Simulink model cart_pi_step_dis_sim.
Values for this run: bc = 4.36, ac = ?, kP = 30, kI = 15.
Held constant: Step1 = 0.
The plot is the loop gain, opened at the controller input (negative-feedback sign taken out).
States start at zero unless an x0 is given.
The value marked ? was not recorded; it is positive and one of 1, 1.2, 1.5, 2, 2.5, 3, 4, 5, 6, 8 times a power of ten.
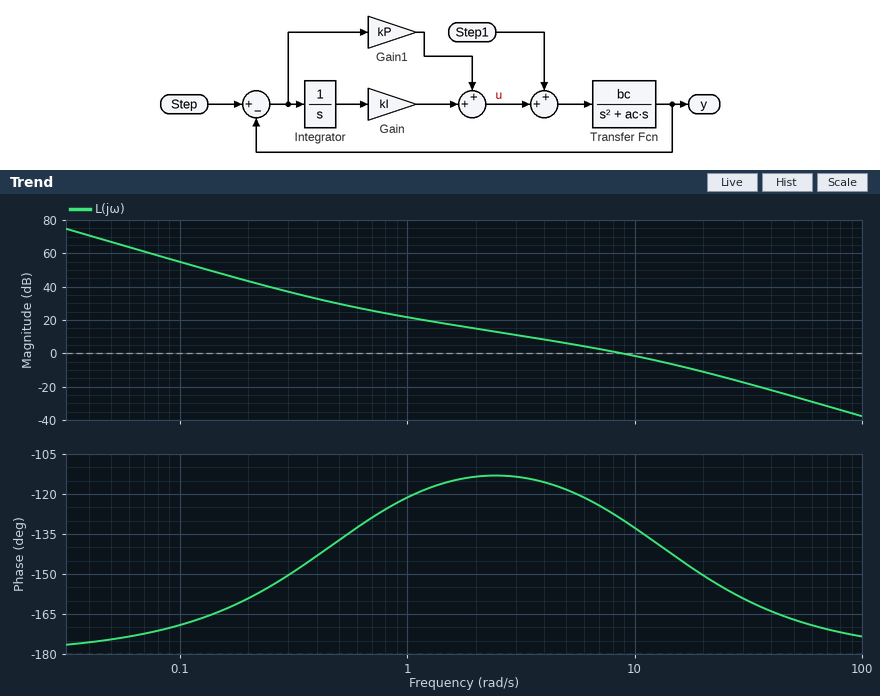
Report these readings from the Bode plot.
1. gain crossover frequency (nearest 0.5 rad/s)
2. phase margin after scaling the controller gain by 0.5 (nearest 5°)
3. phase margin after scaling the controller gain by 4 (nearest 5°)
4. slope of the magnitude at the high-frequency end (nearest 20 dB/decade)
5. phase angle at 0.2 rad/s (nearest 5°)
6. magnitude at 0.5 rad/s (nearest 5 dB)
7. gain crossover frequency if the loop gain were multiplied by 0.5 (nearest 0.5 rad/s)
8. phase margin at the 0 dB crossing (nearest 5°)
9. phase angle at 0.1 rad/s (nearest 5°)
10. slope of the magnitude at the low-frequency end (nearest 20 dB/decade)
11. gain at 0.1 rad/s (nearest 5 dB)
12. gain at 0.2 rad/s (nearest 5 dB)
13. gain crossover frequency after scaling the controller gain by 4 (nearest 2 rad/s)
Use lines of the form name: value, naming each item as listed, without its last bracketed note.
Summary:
gain crossover frequency: 9.0 rad/s
phase margin after scaling the controller gain by 0.5: 60°
phase margin after scaling the controller gain by 4: 30°
slope of the magnitude at the high-frequency end: -40 dB/decade
phase angle at 0.2 rad/s: -160°
magnitude at 0.5 rad/s: 30 dB
gain crossover frequency if the loop gain were multiplied by 0.5: 5.0 rad/s
phase margin at the 0 dB crossing: 50°
phase angle at 0.1 rad/s: -170°
slope of the magnitude at the low-frequency end: -40 dB/decade
gain at 0.1 rad/s: 55 dB
gain at 0.2 rad/s: 45 dB
gain crossover frequency after scaling the controller gain by 4: 22 rad/s
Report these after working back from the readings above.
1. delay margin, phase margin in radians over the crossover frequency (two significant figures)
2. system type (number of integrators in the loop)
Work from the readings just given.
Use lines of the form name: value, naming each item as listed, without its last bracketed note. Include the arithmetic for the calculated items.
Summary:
delay margin, phase margin in radians over the crossover frequency: 50 × π / 180 / 9 = 0.097 s
system type: 2
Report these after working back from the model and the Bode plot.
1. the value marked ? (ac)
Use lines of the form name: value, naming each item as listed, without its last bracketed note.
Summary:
the value marked ?: 12
